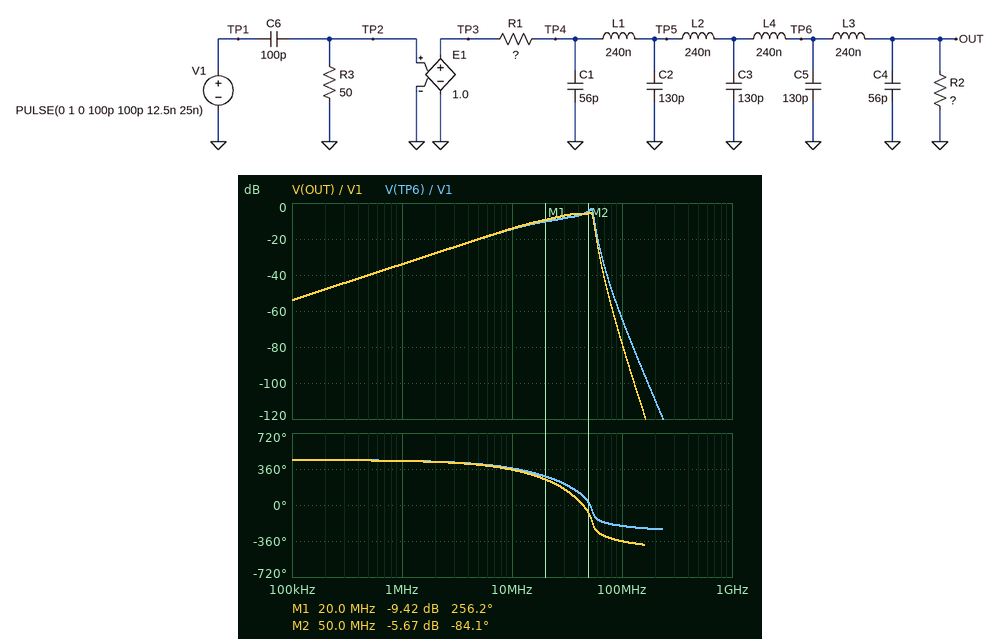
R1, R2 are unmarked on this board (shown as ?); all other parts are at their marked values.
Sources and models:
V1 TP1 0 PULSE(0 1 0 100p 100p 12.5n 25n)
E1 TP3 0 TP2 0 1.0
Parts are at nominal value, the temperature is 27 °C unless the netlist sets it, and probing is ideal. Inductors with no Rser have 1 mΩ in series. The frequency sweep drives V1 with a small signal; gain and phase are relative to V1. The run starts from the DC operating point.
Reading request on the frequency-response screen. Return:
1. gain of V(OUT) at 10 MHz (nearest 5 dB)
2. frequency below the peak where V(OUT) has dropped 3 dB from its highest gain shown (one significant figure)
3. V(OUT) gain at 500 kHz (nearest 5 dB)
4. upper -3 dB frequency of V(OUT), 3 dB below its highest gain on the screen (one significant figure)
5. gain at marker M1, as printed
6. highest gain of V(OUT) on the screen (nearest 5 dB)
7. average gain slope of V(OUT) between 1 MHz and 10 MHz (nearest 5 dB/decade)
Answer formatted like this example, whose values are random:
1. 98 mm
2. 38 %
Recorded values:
1. -15 dB
2. 20 MHz
3. -40 dB
4. 50 MHz
5. -9.42 dB
6. -5 dB
7. 20 dB/decade
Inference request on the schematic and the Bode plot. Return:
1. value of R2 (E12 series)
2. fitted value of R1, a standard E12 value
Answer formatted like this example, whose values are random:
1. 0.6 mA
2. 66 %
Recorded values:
1. 68 Ω
2. 39 Ω
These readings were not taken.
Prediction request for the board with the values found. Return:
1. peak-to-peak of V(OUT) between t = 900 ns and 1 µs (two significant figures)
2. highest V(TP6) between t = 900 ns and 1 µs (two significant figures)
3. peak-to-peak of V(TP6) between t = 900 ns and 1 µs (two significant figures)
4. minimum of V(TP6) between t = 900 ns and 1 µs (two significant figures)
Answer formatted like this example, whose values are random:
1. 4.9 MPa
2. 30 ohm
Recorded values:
1. 630 mV
2. 280 mV
3. 570 mV
4. -280 mV
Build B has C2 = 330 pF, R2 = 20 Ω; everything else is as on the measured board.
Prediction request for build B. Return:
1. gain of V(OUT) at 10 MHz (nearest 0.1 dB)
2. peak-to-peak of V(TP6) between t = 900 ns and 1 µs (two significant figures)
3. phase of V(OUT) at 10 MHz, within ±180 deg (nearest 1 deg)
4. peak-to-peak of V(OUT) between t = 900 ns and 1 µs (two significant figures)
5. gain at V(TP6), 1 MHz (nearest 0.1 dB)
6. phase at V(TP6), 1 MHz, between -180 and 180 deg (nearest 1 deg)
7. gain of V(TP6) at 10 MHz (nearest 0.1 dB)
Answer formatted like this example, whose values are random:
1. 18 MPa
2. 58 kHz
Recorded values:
1. -19.8 dB
2. 310 mV
3. -26 deg
4. 100 mV
5. -39.4 dB
6. 83 deg
7. -18.2 dB
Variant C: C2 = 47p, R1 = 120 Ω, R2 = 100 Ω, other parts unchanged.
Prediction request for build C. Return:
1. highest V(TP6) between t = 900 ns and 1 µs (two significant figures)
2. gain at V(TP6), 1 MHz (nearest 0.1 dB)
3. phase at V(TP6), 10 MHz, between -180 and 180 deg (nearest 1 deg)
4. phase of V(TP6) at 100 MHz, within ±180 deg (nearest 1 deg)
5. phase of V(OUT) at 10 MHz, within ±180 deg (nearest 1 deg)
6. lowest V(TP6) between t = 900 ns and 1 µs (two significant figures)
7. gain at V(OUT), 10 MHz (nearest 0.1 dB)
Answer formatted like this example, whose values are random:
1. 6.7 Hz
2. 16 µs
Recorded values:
1. 140 mV
2. -37.0 dB
3. 5 deg
4. 126 deg
5. -4 deg
6. -140 mV
7. -19.8 dB
